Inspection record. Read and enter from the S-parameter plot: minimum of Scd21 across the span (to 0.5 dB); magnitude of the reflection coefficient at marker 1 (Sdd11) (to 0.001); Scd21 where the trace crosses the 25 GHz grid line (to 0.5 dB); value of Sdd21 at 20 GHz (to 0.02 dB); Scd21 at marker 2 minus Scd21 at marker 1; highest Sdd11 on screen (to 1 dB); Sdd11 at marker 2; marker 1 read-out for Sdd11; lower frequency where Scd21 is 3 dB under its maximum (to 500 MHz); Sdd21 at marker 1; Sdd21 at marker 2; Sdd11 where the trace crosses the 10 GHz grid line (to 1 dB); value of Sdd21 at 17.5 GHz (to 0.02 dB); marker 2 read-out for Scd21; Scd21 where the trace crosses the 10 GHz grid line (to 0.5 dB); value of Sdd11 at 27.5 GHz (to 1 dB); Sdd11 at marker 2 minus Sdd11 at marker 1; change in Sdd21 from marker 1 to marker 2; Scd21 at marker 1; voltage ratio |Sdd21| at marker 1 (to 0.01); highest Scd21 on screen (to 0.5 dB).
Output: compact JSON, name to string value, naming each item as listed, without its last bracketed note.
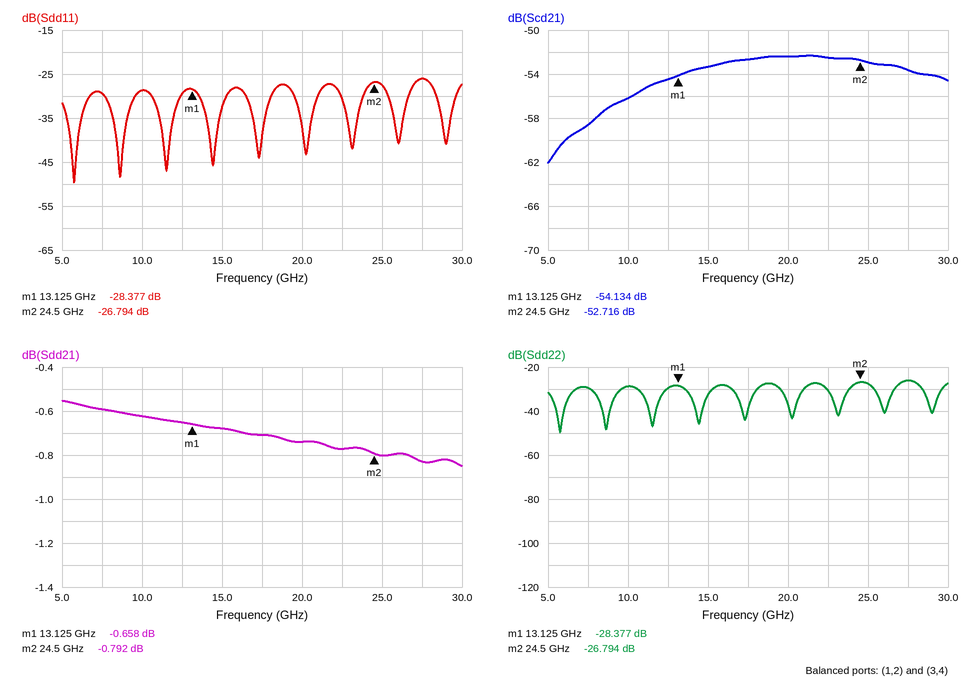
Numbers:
{"minimum of Scd21 across the span": "-62.0 dB", "magnitude of the reflection coefficient at marker 1 (Sdd11)": "0.038", "Scd21 where the trace crosses the 25 GHz grid line": "-53.0 dB", "value of Sdd21 at 20 GHz": "-0.74 dB", "Scd21 at marker 2 minus Scd21 at marker 1": "1.418 dB", "highest Sdd11 on screen": "-26 dB", "Sdd11 at marker 2": "-26.794 dB", "marker 1 read-out for Sdd11": "-28.377 dB", "lower frequency where Scd21 is 3 dB under its maximum": "11.0 GHz", "Sdd21 at marker 1": "-0.658 dB", "Sdd21 at marker 2": "-0.792 dB", "Sdd11 where the trace crosses the 10 GHz grid line": "-29 dB", "value of Sdd21 at 17.5 GHz": "-0.70 dB", "marker 2 read-out for Scd21": "-52.716 dB", "Scd21 where the trace crosses the 10 GHz grid line": "-56.0 dB", "value of Sdd11 at 27.5 GHz": "-26 dB", "Sdd11 at marker 2 minus Sdd11 at marker 1": "1.583 dB", "change in Sdd21 from marker 1 to marker 2": "-0.134 dB", "Scd21 at marker 1": "-54.134 dB", "voltage ratio |Sdd21| at marker 1": "0.93", "highest Scd21 on screen": "-52.5 dB"}
